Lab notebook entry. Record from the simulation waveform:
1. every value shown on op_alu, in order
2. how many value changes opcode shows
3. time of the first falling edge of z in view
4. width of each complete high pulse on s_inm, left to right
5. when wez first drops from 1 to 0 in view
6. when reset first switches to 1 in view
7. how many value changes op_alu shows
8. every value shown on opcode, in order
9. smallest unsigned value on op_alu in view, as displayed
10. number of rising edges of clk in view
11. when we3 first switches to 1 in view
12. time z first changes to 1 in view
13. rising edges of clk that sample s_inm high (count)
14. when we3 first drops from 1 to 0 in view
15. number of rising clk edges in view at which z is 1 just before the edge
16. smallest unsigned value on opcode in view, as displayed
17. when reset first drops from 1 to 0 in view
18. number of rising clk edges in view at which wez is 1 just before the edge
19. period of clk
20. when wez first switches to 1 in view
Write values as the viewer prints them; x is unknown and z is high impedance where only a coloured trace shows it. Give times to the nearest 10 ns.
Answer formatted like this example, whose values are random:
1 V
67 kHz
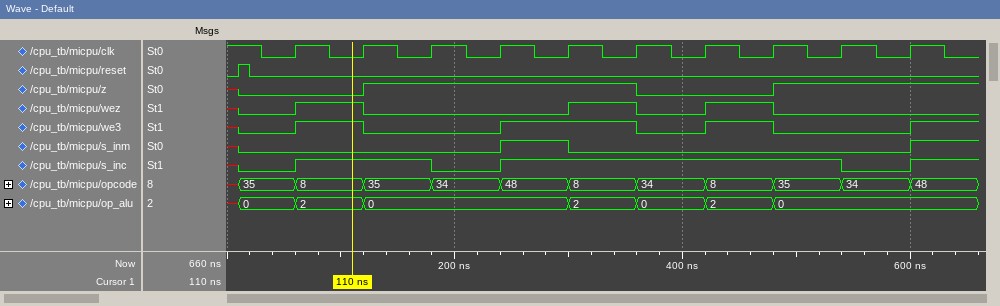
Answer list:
x, 0, 2, 0, 2, 0, 2, 0
11
360 ns
60 ns
120 ns
10 ns
7
x, 35, 8, 35, 34, 48, 8, 34, 8, 35, 34, 48
0
10
60 ns
120 ns
1
120 ns
6
8
20 ns
3
60 ns
60 ns
